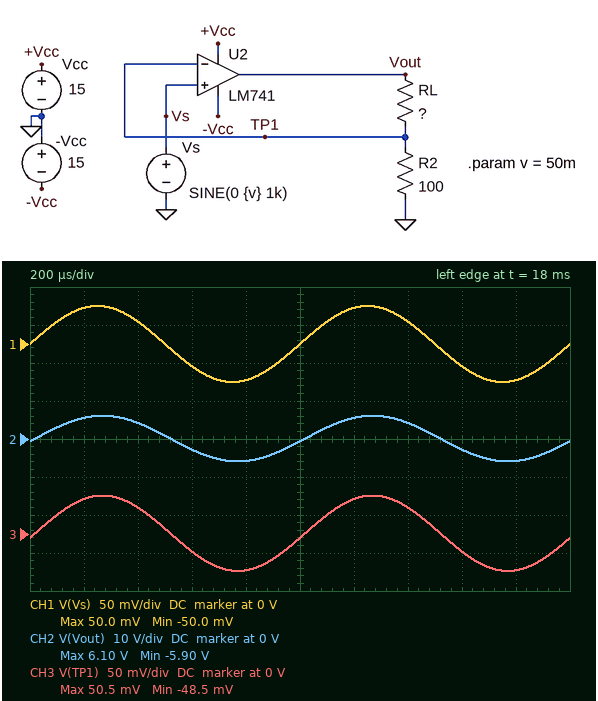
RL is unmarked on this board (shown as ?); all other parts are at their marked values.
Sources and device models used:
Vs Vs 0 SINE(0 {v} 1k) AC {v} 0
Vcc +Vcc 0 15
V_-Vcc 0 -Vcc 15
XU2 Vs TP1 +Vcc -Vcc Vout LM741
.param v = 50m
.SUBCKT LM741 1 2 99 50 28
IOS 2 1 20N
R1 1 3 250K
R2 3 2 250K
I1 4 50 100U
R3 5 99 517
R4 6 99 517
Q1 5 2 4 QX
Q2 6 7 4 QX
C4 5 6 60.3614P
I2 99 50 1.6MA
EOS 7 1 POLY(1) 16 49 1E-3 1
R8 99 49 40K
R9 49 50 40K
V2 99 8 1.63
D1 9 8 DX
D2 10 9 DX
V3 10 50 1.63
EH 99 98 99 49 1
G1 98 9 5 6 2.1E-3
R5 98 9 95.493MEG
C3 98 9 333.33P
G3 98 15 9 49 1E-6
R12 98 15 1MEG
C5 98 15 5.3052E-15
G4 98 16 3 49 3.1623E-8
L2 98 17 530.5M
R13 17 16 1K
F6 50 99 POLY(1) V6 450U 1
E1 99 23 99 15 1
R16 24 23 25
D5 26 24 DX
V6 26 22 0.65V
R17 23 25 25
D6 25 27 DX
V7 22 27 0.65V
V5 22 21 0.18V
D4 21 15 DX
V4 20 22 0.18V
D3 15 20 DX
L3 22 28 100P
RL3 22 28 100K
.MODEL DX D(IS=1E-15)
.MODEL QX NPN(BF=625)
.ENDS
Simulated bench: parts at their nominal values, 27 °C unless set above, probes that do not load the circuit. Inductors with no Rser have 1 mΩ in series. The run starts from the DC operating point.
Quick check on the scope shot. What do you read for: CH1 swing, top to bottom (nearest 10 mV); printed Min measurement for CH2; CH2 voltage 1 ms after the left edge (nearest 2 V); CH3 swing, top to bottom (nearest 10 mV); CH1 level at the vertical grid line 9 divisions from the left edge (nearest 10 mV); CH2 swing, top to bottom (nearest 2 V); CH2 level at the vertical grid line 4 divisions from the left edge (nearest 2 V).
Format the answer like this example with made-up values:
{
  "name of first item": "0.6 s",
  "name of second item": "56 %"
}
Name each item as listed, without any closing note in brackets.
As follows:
{
  "CH1 swing, top to bottom": "100 mV",
  "printed Min measurement for CH2": "-5.90 V",
  "CH2 voltage 1 ms after the left edge": "0 V",
  "CH3 swing, top to bottom": "100 mV",
  "CH1 level at the vertical grid line 9 divisions from the left edge": "-50 mV",
  "CH2 swing, top to bottom": "12 V",
  "CH2 level at the vertical grid line 4 divisions from the left edge": "-6 V"
}
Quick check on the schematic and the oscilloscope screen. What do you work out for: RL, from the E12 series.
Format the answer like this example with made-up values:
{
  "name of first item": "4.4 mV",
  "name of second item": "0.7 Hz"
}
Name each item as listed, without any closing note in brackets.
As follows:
{
  "RL, from the E12 series": "12 kΩ"
}
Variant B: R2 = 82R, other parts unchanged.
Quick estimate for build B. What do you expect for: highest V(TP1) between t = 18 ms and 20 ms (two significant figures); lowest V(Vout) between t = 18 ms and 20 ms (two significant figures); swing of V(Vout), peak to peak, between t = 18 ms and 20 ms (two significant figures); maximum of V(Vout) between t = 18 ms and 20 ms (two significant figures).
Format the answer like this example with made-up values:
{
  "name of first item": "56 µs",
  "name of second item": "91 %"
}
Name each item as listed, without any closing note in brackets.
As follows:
{
  "highest V(TP1) between t = 18 ms and 20 ms": "50 mV",
  "lowest V(Vout) between t = 18 ms and 20 ms": "-7.1 V",
  "swing of V(Vout), peak to peak, between t = 18 ms and 20 ms": "15 V",
  "maximum of V(Vout) between t = 18 ms and 20 ms": "7.4 V"
}
